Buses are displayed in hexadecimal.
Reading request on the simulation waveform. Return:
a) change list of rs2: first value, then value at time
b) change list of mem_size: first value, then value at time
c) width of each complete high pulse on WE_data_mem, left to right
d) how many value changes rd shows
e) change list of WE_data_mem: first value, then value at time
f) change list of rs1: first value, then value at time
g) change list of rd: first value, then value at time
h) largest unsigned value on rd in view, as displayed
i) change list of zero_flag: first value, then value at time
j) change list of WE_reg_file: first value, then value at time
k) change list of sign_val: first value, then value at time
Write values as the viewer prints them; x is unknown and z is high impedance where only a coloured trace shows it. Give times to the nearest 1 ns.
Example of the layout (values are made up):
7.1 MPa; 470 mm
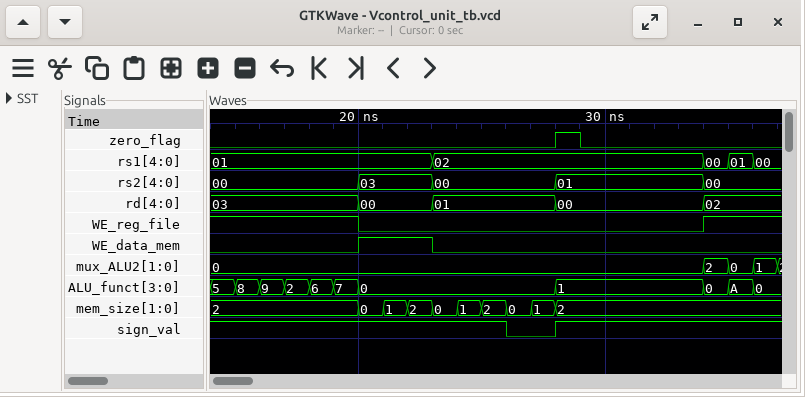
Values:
00, 03 at 20 ns, 00 at 23 ns, 01 at 28 ns, 00 at 34 ns; 2, 0 at 20 ns, 1 at 21 ns, 2 at 22 ns, 0 at 23 ns, 1 at 24 ns, 2 at 25 ns, 0 at 26 ns, 1 at 27 ns, 2 at 28 ns; 3 ns; 4; 0, 1 at 20 ns, 0 at 23 ns; 01, 02 at 23 ns, 00 at 34 ns, 01 at 35 ns, 00 at 36 ns; 03, 00 at 20 ns, 01 at 23 ns, 00 at 28 ns, 02 at 34 ns; 03; 0, 1 at 28 ns, 0 at 29 ns; 1, 0 at 20 ns, 1 at 34 ns; 1, 0 at 26 ns, 1 at 28 ns
